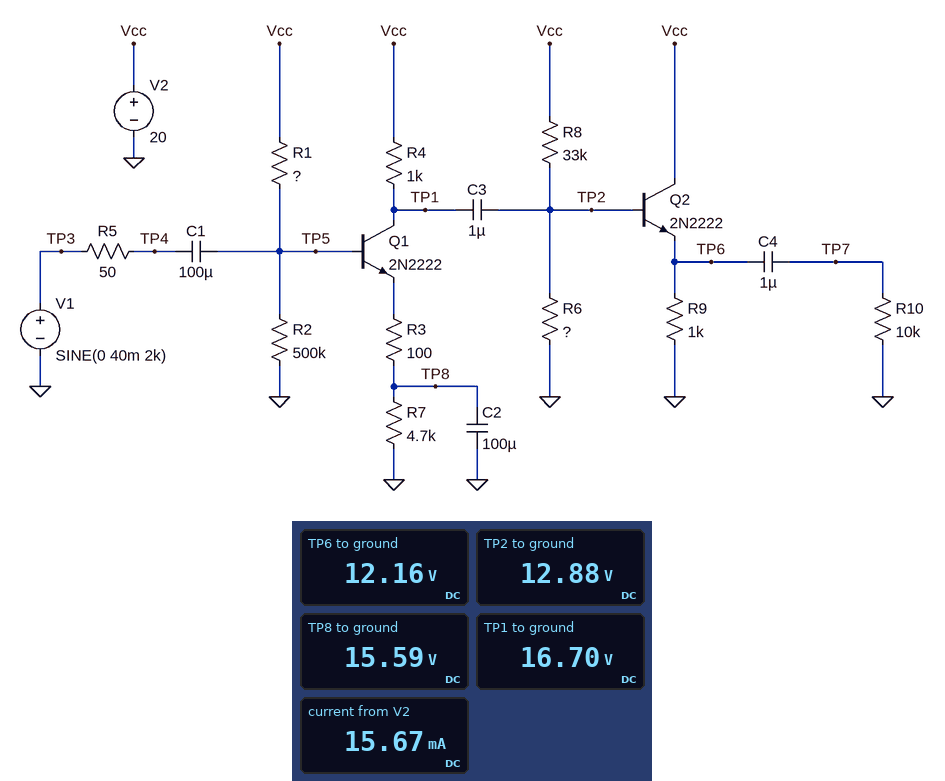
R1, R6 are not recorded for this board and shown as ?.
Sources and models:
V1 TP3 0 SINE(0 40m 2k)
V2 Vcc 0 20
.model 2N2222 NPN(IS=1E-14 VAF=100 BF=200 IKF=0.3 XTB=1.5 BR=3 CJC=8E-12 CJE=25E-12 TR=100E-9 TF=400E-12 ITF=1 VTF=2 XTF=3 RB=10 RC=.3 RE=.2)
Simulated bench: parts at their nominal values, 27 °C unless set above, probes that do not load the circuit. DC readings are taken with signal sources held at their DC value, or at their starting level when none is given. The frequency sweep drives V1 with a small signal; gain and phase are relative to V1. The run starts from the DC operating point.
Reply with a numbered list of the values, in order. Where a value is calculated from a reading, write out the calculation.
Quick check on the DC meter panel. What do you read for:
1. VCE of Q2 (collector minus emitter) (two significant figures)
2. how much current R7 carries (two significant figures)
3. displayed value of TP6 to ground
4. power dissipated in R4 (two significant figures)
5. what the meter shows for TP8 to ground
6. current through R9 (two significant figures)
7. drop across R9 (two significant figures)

1. 20 V - 12.16 V = 7.8 V
2. (15.59 V) / 4.7 kΩ = 3.3 mA
3. 12.16 V
4. (20 V - 16.7 V)^2 / 1 kΩ = 11 mW
5. 15.59 V
6. (12.16 V) / 1 kΩ = 12 mA
7. 12.16 V = 12 V
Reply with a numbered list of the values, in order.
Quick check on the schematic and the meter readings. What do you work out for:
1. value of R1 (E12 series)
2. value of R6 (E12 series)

1. 68 kΩ
2. 82 kΩ
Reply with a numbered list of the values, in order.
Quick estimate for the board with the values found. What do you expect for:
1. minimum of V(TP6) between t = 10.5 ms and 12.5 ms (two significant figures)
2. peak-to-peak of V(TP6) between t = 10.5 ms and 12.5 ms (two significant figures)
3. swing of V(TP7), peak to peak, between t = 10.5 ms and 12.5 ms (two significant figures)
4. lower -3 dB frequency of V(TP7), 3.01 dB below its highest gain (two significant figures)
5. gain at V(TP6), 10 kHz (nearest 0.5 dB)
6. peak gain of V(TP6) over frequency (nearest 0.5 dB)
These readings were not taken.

1. 12 V
2. 700 mV
3. 700 mV
4. 26 Hz
5. 19.0 dB
6. 19.0 dB
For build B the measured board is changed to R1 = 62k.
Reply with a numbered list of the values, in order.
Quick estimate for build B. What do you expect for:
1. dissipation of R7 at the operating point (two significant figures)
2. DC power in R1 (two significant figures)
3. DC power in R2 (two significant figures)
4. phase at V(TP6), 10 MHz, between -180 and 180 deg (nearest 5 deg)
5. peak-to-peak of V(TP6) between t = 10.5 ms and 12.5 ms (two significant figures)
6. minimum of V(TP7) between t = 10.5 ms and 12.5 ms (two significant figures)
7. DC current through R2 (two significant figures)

1. 53 mW
2. 160 µW
3. 570 µW
4. 125 deg
5. 670 mV
6. -330 mV
7. 34 µA
